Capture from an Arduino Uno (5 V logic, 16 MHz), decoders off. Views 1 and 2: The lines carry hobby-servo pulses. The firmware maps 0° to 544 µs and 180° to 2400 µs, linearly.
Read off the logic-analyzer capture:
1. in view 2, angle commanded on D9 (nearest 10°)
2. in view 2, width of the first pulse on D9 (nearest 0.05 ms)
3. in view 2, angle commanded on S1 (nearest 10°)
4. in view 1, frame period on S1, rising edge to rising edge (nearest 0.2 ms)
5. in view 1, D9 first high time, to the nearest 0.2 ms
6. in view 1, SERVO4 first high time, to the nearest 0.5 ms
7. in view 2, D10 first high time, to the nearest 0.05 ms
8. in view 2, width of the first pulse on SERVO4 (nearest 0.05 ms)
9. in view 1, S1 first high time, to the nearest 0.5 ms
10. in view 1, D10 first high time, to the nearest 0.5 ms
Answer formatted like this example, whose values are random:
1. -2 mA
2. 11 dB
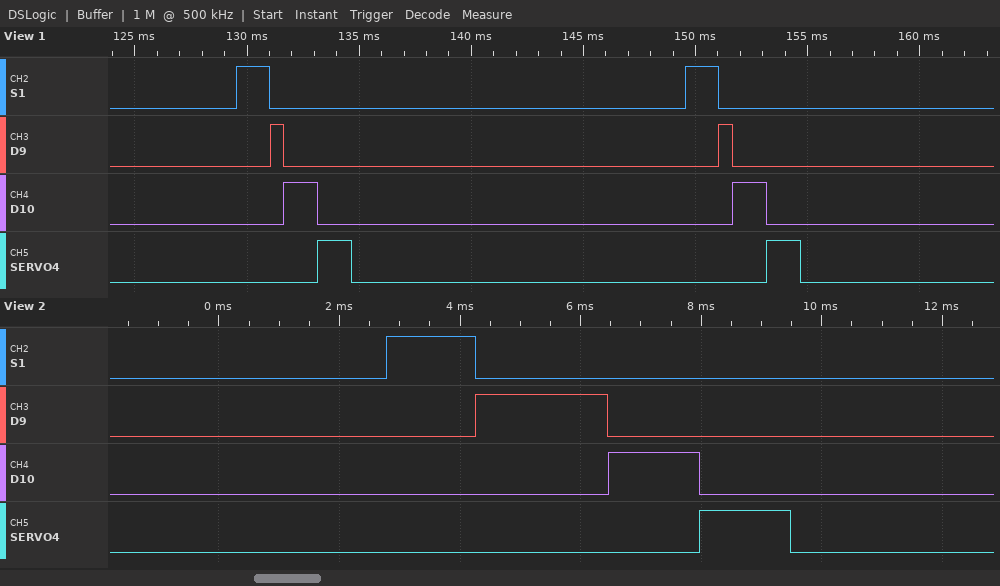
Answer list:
1. 160°
2. 2.20 ms
3. 90°
4. 20.0 ms
5. 0.6 ms
6. 1.5 ms
7. 1.50 ms
8. 1.50 ms
9. 1.5 ms
10. 1.5 ms
